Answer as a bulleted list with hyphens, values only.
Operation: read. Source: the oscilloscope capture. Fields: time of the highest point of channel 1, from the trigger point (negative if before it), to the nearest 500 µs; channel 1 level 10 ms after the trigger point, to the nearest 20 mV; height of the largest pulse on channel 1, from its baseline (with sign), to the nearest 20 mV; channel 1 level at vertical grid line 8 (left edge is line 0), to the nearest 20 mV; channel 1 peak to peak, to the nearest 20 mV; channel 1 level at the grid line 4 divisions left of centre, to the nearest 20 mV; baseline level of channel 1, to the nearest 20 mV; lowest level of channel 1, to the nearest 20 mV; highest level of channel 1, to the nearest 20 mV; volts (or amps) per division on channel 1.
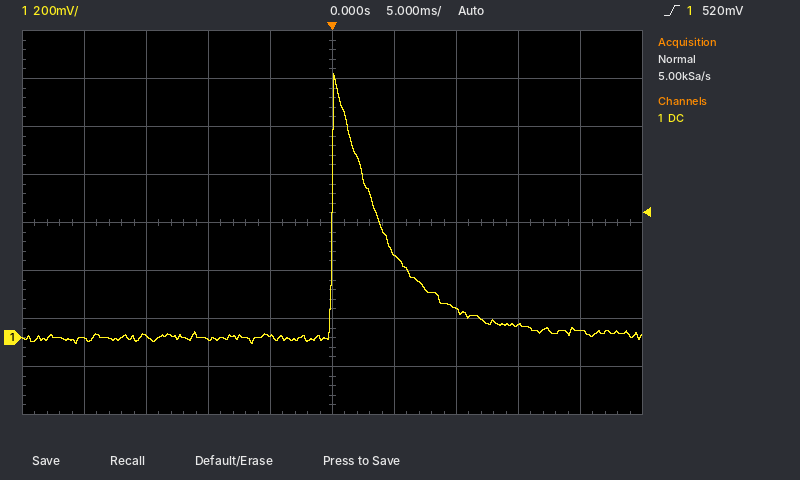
- 0.0 ms
- 120 mV
- +1.10 V
- 60 mV
- 1.12 V
- 0 mV
- 0 mV
- -20 mV
- 1.10 V
- 200 mV
